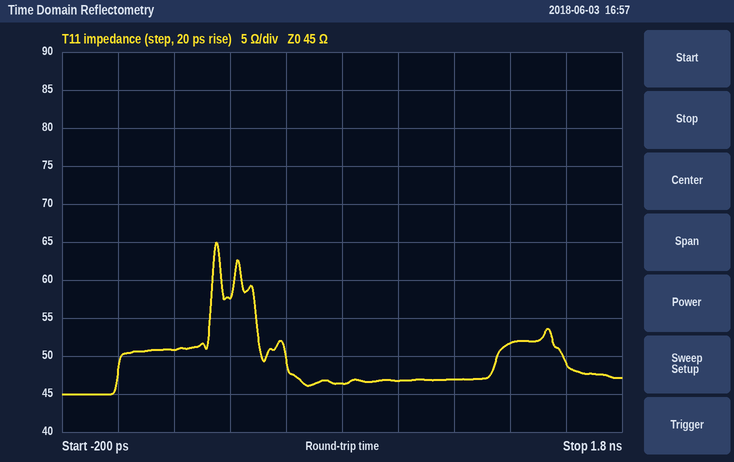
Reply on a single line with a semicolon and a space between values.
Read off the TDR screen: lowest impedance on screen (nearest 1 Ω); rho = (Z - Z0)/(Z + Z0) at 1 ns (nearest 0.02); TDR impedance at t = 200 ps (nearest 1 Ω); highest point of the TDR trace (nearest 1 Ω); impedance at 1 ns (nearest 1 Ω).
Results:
45 Ω; +0.02; 51 Ω; 65 Ω; 47 Ω
